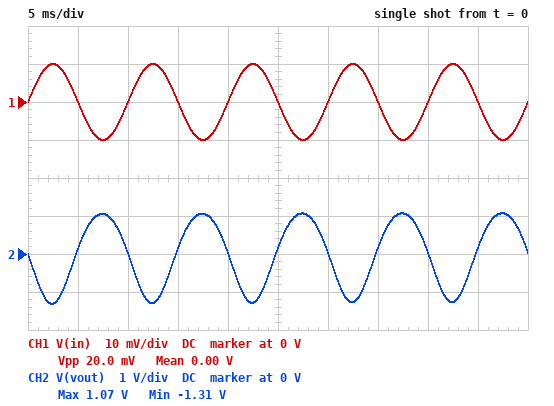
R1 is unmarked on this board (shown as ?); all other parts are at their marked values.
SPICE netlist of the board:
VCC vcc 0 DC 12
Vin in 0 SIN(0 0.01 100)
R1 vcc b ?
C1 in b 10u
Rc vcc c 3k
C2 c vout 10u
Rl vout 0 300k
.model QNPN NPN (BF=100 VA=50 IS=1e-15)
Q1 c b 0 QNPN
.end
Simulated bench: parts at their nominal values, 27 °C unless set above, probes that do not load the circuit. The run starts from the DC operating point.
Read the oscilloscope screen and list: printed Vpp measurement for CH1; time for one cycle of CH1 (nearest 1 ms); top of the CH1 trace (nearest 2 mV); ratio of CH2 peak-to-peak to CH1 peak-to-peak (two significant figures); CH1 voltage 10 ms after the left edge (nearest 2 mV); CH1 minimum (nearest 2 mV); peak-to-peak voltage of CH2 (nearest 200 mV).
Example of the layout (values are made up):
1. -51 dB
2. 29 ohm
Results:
1. 20.0 mV
2. 10 ms
3. 10 mV
4. 120
5. 0 V
6. -10 mV
7. 2.4 V
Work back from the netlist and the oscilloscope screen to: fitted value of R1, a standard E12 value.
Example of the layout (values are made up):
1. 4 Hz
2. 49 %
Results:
1. 1.2 MΩ
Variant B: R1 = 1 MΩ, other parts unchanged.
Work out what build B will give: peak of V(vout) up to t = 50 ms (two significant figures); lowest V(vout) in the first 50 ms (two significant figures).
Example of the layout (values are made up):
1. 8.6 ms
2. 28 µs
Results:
1. 1.3 V
2. -1.5 V
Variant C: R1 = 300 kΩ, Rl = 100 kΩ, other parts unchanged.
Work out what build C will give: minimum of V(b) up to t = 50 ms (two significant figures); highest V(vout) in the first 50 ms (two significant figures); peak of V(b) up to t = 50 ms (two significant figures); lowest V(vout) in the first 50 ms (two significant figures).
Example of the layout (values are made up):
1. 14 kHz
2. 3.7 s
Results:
1. 730 mV
2. 4.2 V
3. 750 mV
4. -700 mV
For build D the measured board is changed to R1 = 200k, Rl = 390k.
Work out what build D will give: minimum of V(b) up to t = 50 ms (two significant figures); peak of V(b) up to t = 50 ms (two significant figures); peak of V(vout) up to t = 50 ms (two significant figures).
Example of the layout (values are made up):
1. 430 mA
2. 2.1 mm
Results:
1. 740 mV
2. 750 mV
3. 3.2 V
